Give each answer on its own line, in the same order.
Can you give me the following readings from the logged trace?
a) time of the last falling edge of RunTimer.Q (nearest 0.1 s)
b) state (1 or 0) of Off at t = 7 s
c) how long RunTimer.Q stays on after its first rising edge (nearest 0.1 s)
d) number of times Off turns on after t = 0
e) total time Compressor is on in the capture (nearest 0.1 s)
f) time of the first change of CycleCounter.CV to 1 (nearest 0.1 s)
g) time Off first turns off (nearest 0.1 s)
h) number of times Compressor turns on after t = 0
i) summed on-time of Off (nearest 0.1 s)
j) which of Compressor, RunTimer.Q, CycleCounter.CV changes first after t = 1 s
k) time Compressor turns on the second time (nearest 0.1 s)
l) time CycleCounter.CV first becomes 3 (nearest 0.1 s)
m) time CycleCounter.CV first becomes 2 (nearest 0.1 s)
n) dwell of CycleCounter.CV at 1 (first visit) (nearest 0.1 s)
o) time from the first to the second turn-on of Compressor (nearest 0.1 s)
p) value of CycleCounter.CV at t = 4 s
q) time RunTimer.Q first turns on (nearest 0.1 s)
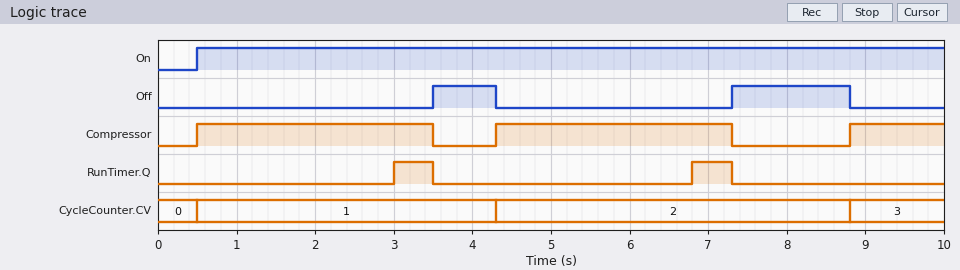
7.3 s
0
0.5 s
2
7.2 s
0.5 s
4.3 s
3
2.3 s
RunTimer.Q
4.3 s
8.8 s
4.3 s
3.8 s
3.8 s
1
3.0 s
